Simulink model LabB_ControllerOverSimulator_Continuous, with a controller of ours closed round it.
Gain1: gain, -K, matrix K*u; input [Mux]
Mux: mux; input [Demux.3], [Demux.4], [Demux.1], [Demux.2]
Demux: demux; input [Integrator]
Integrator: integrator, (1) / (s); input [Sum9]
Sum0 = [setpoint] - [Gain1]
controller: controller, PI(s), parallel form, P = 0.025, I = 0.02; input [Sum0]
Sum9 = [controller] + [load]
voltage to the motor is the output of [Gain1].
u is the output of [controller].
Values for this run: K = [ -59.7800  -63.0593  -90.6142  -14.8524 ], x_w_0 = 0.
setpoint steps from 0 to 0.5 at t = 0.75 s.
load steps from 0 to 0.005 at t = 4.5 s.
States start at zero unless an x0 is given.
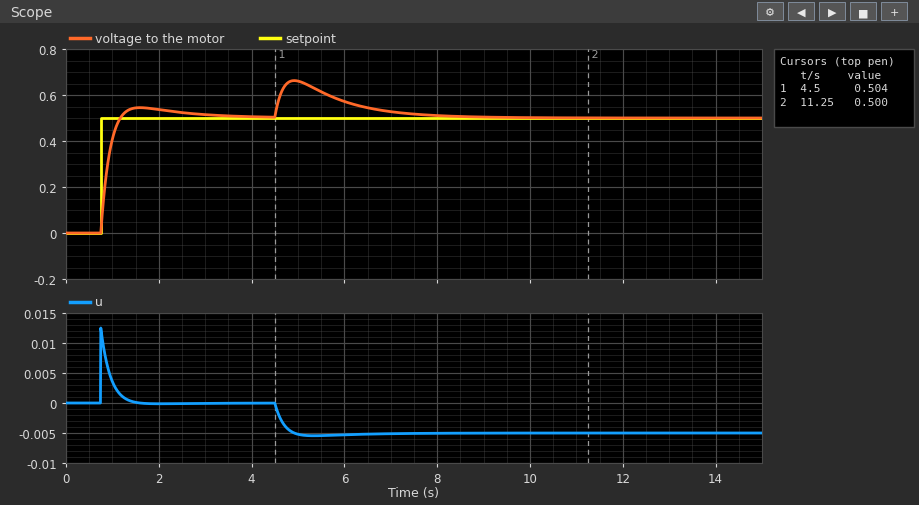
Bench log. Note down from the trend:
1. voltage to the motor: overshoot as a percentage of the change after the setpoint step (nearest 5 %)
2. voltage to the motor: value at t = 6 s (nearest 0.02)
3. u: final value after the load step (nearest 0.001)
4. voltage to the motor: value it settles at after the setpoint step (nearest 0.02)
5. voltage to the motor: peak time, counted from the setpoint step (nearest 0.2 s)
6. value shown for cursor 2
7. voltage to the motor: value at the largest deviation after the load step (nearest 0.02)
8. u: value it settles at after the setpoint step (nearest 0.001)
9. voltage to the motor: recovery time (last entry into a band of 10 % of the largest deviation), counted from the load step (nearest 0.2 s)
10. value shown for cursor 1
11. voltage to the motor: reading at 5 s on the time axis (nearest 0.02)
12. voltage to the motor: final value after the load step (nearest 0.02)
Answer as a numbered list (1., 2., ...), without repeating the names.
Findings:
1. 10 %
2. 0.58
3. -0.005
4. 0.50
5. 0.8 s
6. 0.500
7. 0.66
8. 0.000
9. 3.0 s
10. 0.504
11. 0.66
12. 0.50
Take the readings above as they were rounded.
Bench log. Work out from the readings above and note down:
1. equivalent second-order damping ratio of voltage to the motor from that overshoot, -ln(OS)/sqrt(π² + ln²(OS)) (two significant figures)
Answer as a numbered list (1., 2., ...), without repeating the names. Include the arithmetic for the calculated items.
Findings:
1. ln(0.1) = -2.303; 2.303 / sqrt(9.870 + 5.302) = 0.59
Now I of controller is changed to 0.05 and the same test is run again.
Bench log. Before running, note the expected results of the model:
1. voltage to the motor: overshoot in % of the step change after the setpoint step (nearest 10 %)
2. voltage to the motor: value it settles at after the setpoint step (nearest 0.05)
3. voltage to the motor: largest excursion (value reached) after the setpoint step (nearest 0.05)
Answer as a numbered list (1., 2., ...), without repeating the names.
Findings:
1. 20 %
2. 0.50
3. 0.60
